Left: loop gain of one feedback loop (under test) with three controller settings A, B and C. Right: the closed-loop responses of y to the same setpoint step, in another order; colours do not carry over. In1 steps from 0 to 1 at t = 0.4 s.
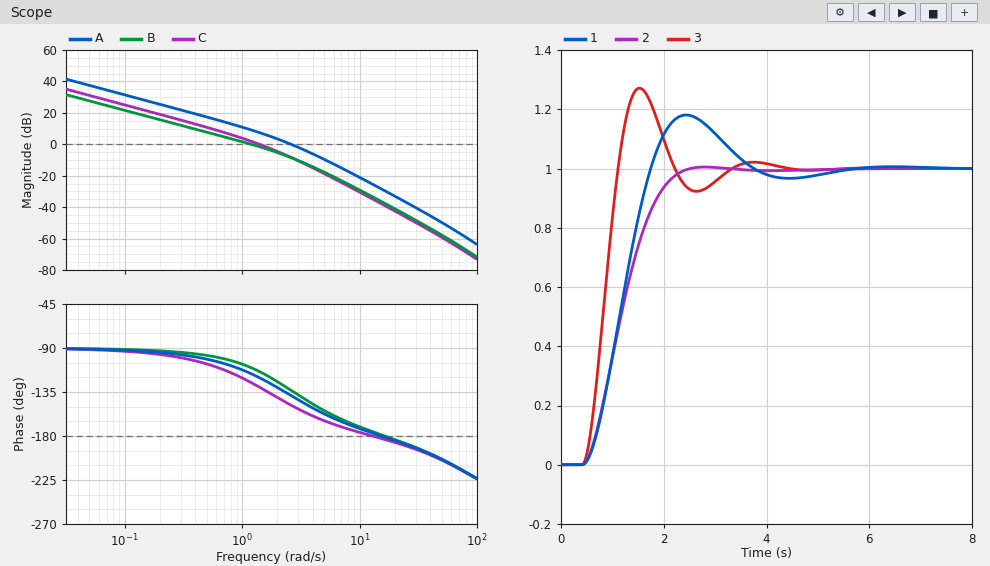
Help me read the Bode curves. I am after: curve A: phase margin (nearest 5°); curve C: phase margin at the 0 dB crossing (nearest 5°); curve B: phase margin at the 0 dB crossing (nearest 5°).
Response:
40°
50°
70°
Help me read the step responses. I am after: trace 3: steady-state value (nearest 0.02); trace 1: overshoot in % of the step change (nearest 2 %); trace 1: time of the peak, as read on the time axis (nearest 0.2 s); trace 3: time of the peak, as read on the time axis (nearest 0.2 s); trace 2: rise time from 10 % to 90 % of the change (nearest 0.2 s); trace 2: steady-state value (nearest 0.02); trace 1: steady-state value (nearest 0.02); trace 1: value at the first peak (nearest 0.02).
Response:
1.00
18 %
2.4 s
1.6 s
1.2 s
1.00
1.00
1.18
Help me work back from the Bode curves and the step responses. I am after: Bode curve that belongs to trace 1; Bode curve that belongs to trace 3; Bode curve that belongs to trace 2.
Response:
C
A
B
